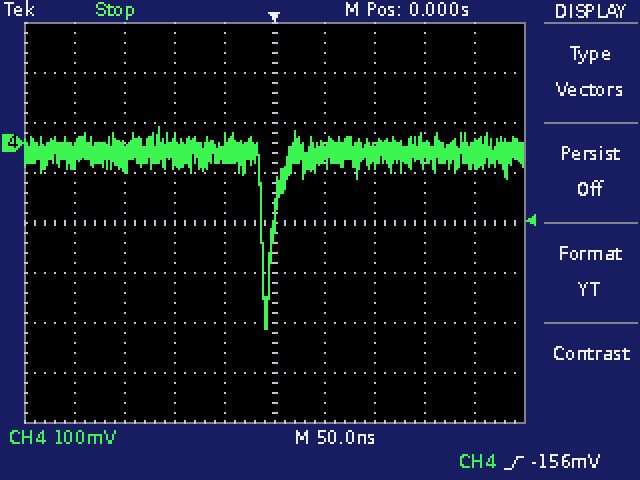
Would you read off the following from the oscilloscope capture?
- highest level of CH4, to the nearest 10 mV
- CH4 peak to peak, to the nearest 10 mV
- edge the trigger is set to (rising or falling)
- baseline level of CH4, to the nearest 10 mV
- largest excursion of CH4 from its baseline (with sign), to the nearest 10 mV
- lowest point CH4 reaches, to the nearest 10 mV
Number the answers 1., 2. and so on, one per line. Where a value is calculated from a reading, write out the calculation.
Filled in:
1. 30 mV
2. 30 mV − (-370 mV) = 400 mV
3. rising
4. -20 mV
5. -370 mV − (-20 mV) = -350 mV
6. -370 mV
